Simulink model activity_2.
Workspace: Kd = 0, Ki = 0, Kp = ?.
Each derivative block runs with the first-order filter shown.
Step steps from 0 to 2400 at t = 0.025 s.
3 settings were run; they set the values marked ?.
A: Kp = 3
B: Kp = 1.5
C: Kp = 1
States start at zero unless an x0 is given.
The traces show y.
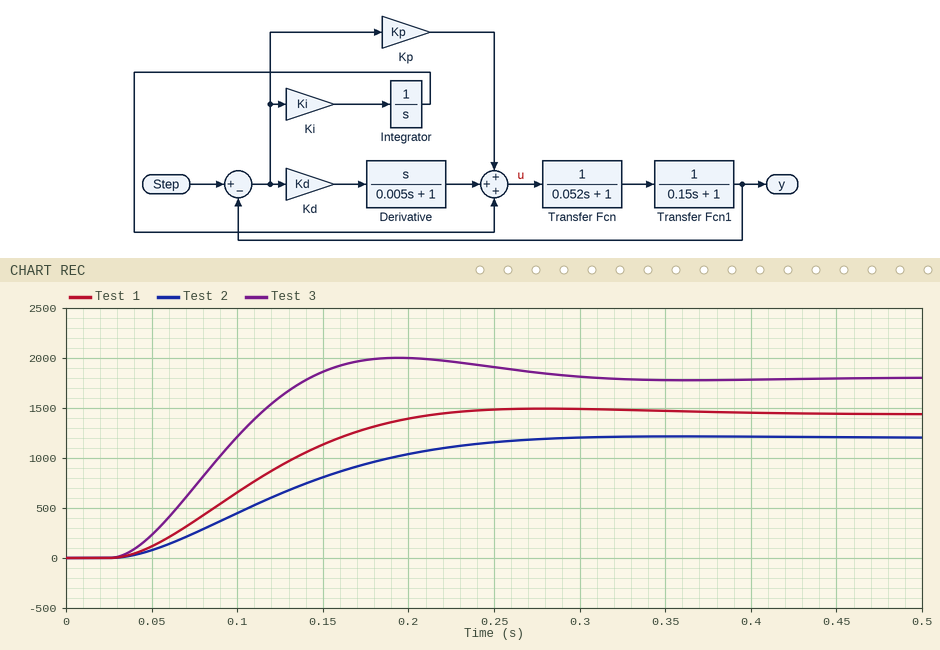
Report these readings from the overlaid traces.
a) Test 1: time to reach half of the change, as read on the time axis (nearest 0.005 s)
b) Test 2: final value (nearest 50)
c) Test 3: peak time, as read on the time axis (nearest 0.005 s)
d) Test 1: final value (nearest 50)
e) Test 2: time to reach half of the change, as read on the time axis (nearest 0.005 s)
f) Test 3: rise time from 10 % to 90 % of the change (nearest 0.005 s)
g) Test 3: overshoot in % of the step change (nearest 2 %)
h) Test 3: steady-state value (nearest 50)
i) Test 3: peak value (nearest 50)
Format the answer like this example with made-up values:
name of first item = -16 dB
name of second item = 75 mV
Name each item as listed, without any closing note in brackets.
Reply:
Test 1: time to reach half of the change, as read on the time axis = 0.105 s
Test 2: final value = 1200
Test 3: peak time, as read on the time axis = 0.195 s
Test 1: final value = 1450
Test 2: time to reach half of the change, as read on the time axis = 0.120 s
Test 3: rise time from 10 % to 90 % of the change = 0.080 s
Test 3: overshoot in % of the step change = 12 %
Test 3: steady-state value = 1800
Test 3: peak value = 2000
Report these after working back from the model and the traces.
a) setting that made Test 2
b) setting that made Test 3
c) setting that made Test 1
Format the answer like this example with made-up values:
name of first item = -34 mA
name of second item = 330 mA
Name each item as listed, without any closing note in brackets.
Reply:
setting that made Test 2 = C
setting that made Test 3 = A
setting that made Test 1 = B
